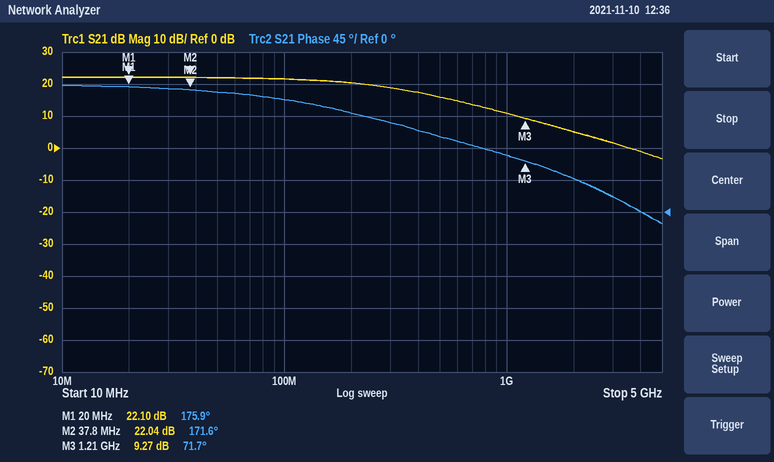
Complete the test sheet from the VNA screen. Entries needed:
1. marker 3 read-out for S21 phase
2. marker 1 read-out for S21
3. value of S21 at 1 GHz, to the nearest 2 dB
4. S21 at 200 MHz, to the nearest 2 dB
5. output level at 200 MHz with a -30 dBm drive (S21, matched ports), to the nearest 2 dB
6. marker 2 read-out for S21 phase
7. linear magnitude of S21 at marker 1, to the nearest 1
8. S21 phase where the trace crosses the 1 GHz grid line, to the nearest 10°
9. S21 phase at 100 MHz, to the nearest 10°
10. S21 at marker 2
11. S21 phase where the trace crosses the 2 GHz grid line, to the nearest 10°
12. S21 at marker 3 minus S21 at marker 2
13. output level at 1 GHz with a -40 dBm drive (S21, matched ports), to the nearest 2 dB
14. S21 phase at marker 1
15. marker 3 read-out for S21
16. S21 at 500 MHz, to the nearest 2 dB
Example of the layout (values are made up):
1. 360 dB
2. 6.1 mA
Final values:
1. 71.7°
2. 22.10 dB
3. 10 dB
4. 20 dB
5. -10 dBm
6. 171.6°
7. 13
8. 80°
9. 160°
10. 22.04 dB
11. 50°
12. -12.77 dB
13. -30 dBm
14. 175.9°
15. 9.27 dB
16. 16 dB
